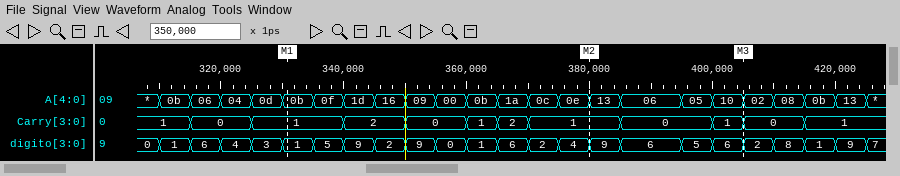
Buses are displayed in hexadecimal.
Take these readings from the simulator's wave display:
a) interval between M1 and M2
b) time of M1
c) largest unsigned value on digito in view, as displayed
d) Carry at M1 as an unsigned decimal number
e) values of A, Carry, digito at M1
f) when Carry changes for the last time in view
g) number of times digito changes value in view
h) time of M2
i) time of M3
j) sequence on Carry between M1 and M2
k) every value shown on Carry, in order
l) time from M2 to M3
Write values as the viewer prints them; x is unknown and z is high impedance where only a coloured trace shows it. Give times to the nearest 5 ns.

50 ns
330 ns
9
1
A=0b, Carry=1, digito=1
415 ns
23
380 ns
405 ns
1, 2, 0, 1, 2, 1
1, 0, 1, 2, 0, 1, 2, 1, 0, 1, 0, 1
25 ns
